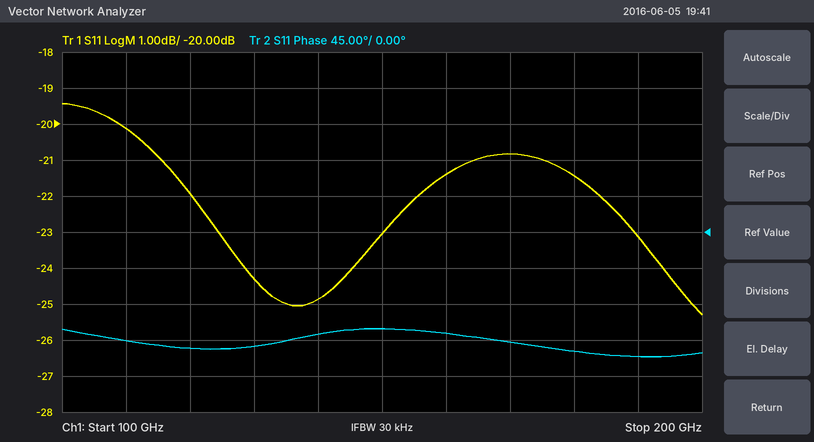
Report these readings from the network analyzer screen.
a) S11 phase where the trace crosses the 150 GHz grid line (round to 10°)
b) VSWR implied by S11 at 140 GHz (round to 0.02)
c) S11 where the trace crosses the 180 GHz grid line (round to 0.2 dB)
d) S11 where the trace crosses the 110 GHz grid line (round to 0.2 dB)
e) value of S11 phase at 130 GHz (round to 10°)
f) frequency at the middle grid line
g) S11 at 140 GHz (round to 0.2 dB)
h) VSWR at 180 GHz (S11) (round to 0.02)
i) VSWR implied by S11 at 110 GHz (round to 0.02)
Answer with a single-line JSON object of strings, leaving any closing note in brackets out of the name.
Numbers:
{"S11 phase where the trace crosses the 150 GHz grid line": "-120°", "VSWR implied by S11 at 140 GHz": "1.12", "S11 where the trace crosses the 180 GHz grid line": "-21.4 dB", "S11 where the trace crosses the 110 GHz grid line": "-20.2 dB", "value of S11 phase at 130 GHz": "-140°", "frequency at the middle grid line": "150 GHz", "S11 at 140 GHz": "-24.8 dB", "VSWR at 180 GHz (S11)": "1.18", "VSWR implied by S11 at 110 GHz": "1.22"}
